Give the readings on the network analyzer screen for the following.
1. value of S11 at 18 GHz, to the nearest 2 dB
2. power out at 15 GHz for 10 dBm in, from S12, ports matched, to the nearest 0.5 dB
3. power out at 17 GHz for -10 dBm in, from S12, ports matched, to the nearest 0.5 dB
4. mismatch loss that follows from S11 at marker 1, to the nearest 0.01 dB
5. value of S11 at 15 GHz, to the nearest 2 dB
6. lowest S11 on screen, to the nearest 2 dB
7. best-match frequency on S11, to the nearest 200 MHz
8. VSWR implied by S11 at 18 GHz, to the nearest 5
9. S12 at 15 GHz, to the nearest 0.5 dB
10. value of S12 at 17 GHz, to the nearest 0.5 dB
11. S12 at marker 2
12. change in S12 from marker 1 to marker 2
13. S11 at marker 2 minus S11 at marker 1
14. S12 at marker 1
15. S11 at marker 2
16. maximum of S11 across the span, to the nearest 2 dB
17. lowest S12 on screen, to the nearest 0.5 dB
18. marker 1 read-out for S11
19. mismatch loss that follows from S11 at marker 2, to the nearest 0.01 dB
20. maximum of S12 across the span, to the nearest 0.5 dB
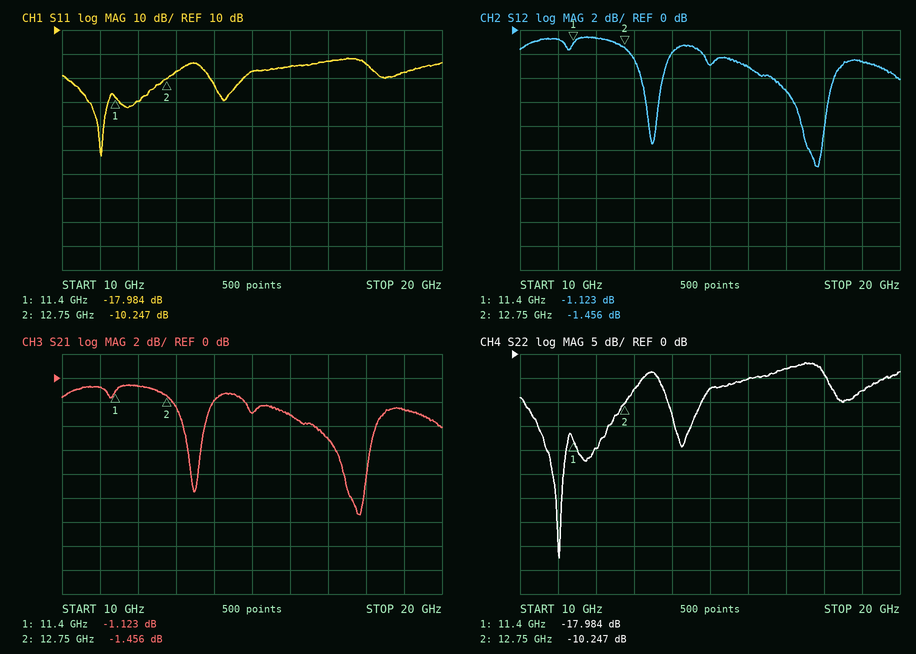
-4 dB
7.0 dBm
-15.0 dBm
0.07 dB
-8 dB
-42 dB
11.0 GHz
5
-3.0 dB
-5.0 dB
-1.456 dB
-0.333 dB
7.737 dB
-1.123 dB
-10.247 dB
-2 dB
-11.5 dB
-17.984 dB
0.43 dB
-0.5 dB
